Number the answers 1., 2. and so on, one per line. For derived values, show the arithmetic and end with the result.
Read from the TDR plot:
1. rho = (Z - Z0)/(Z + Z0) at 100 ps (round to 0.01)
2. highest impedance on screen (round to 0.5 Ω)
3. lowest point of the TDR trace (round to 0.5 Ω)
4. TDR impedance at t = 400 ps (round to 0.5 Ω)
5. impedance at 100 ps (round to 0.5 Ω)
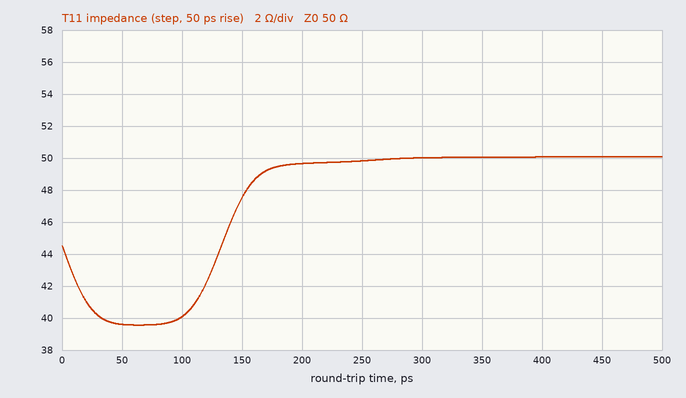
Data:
1. (40 − 50)/(40 + 50) ≈ -0.11
2. 50.0 Ω
3. 39.5 Ω
4. 50.0 Ω
5. 40.0 Ω
